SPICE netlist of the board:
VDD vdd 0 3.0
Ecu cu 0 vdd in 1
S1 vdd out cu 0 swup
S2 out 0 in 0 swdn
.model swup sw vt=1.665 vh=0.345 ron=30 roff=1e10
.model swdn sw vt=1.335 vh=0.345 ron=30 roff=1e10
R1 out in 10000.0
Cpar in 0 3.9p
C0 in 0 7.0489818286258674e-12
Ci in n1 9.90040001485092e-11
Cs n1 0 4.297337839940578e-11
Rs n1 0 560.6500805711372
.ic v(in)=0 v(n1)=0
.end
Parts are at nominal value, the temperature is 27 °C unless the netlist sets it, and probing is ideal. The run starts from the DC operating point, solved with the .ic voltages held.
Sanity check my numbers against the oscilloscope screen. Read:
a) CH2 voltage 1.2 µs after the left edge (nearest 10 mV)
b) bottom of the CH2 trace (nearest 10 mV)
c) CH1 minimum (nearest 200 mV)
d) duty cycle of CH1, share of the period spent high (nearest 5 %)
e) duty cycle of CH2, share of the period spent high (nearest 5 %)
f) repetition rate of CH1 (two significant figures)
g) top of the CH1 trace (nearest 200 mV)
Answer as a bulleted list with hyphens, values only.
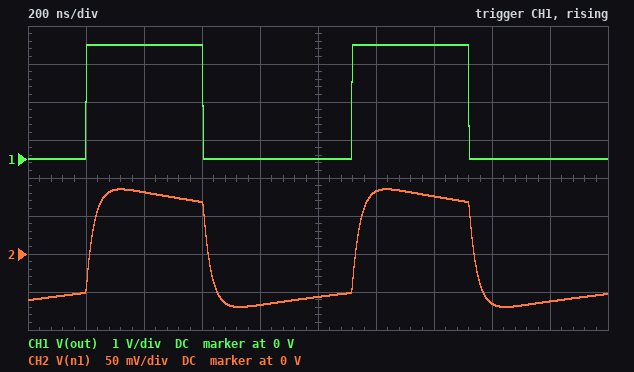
- 80 mV
- -70 mV
- 0 V
- 45 %
- 45 %
- 1.1 MHz
- 3.0 V
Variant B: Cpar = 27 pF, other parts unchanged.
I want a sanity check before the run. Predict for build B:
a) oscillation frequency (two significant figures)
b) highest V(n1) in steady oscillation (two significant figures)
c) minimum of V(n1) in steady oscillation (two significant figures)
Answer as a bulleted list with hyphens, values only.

- 860 kHz
- 71 mV
- -59 mV
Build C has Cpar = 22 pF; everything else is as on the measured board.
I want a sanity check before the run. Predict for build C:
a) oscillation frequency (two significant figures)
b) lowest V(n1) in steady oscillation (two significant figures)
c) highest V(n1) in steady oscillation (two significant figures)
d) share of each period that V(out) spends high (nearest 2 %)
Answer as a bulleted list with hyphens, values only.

- 900 kHz
- -61 mV
- 74 mV
- 44 %
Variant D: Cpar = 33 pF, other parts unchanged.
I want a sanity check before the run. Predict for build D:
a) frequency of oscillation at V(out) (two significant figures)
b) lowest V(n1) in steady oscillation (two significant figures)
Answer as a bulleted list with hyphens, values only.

- 820 kHz
- -56 mV
